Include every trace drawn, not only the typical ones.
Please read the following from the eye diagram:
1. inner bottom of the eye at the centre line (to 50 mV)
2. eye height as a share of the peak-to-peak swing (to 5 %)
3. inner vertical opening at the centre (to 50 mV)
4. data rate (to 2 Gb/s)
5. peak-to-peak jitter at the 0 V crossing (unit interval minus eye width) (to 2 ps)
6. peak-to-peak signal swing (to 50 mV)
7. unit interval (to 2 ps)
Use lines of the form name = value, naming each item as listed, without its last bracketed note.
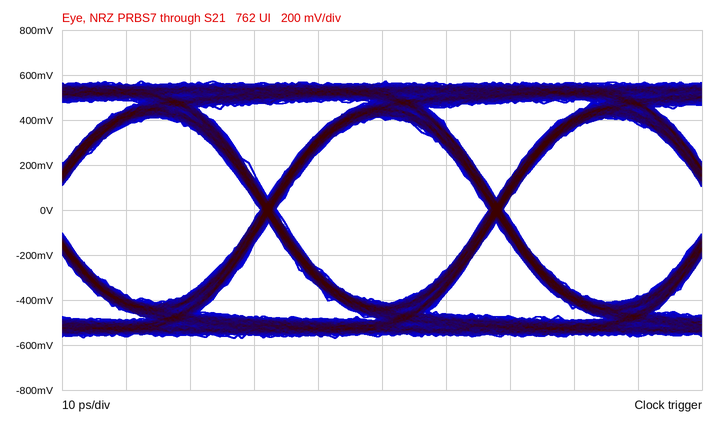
inner bottom of the eye at the centre line = -400 mV
eye height as a share of the peak-to-peak swing = 70 %
inner vertical opening at the centre = 800 mV
data rate = 28 Gb/s
peak-to-peak jitter at the 0 V crossing (unit interval minus eye width) = 2 ps
peak-to-peak signal swing = 1.15 V
unit interval = 36 ps
